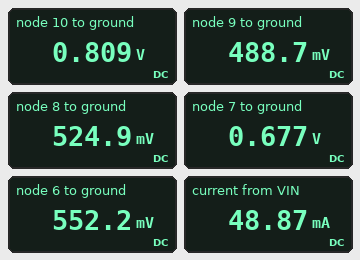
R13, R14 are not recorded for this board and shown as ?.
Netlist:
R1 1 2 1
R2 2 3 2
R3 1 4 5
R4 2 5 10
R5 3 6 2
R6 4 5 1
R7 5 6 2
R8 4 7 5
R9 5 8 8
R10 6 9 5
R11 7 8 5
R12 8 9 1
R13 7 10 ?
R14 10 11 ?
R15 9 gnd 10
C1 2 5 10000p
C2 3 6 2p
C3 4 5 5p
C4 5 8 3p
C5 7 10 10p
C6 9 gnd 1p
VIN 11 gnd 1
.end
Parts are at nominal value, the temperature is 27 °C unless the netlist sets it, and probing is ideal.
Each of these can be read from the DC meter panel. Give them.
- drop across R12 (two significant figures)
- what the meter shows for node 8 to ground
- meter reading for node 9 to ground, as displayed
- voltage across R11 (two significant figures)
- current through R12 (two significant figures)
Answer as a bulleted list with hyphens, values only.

- 36 mV
- 524.9 mV
- 488.7 mV
- 150 mV
- 36 mA
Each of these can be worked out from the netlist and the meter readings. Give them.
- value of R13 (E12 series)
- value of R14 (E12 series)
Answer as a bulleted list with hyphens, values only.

- 2.7 Ω
- 3.9 Ω
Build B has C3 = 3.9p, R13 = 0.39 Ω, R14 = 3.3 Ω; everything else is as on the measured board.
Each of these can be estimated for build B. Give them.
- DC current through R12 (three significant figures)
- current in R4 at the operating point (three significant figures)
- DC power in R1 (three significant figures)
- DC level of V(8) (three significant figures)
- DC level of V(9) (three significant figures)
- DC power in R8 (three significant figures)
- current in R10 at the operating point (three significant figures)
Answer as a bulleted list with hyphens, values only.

- 42.2 mA
- 457 µA
- 13.8 µW
- 612 mV
- 570 mV
- 2.29 mW
- 14.8 mA
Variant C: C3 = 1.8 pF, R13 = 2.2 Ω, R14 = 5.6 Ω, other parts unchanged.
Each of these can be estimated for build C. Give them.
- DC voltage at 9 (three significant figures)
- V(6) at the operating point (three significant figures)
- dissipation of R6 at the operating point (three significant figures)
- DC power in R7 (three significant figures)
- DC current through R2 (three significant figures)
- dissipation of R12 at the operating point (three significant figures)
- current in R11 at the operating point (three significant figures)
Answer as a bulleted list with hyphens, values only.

- 462 mV
- 522 mV
- 206 µW
- 148 µW
- 3.38 mA
- 1.17 mW
- 28.8 mA
